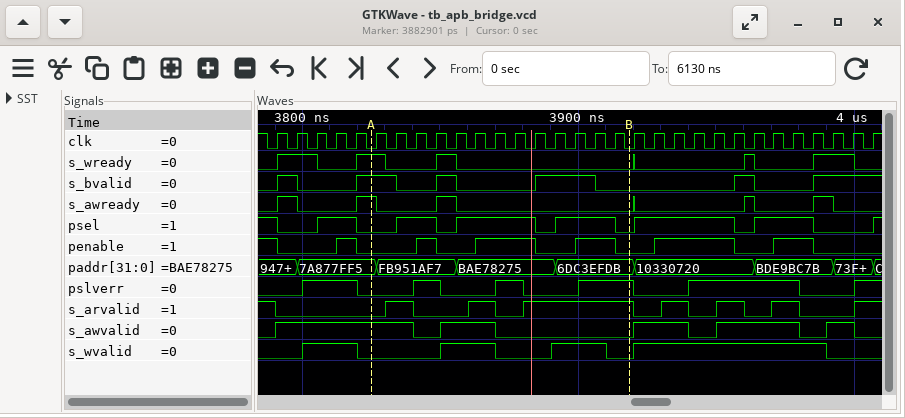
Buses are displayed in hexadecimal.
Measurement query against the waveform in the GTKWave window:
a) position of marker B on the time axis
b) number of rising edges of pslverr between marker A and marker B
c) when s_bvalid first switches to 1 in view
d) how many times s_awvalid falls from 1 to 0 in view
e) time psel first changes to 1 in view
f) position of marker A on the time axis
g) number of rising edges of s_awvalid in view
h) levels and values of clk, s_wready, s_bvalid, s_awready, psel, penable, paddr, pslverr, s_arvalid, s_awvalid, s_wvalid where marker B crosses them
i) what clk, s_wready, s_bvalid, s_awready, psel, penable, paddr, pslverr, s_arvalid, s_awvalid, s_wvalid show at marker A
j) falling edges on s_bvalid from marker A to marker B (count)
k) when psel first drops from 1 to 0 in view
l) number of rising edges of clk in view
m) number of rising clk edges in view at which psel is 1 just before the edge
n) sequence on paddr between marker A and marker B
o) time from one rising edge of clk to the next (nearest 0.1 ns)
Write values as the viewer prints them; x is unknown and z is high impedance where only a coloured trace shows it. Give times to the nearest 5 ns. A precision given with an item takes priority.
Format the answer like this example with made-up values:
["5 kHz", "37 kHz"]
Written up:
["3920 ns", "3", "3790 ns", "5", "3805 ns", "3825 ns", "5", "clk=0, s_wready=0, s_bvalid=0, s_awready=0, psel=0, penable=0, paddr=6DC3EFDB, pslverr=1, s_arvalid=1, s_awvalid=0, s_wvalid=0", "clk=0, s_wready=1, s_bvalid=1, s_awready=1, psel=0, penable=0, paddr=7A877FF5, pslverr=0, s_arvalid=0, s_awvalid=1, s_wvalid=0", "3", "3790 ns", "31", "20", "7A877FF5, FB951AF7, BAE78275, 6DC3EFDB", "7.2 ns"]
